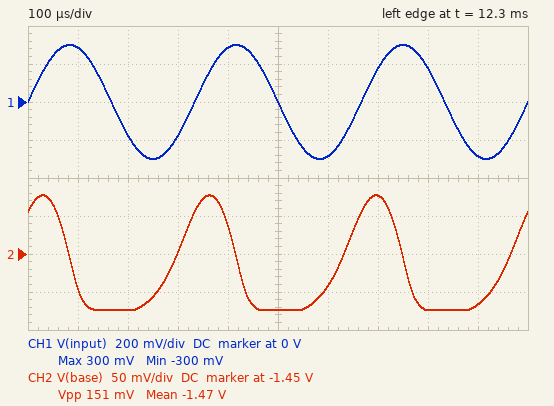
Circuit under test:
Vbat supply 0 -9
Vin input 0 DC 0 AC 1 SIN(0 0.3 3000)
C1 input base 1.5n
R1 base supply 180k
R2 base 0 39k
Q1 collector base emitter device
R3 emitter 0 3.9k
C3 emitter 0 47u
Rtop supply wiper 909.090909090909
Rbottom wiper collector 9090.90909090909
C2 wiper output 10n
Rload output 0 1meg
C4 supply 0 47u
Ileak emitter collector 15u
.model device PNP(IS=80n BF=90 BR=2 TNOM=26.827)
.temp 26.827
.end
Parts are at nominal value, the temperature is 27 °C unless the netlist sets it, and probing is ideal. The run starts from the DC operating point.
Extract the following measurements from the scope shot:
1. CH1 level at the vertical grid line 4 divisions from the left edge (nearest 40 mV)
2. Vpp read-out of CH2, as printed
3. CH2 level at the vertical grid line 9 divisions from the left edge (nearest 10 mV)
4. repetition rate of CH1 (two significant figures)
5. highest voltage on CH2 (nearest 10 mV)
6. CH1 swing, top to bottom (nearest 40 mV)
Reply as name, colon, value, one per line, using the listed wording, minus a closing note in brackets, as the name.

CH1 level at the vertical grid line 4 divisions from the left edge: 280 mV
Vpp read-out of CH2, as printed: 151 mV
CH2 level at the vertical grid line 9 divisions from the left edge: -1.52 V
repetition rate of CH1: 3.0 kHz
highest voltage on CH2: -1.37 V
CH1 swing, top to bottom: 600 mV
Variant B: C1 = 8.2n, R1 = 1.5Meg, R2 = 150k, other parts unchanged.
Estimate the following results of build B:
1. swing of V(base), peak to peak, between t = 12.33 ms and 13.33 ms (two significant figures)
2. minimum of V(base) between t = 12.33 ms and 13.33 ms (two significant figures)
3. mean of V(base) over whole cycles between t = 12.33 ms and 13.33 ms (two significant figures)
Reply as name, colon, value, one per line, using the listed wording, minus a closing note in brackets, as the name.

swing of V(base), peak to peak, between t = 12.33 ms and 13.33 ms: 560 mV
minimum of V(base) between t = 12.33 ms and 13.33 ms: -730 mV
mean of V(base) over whole cycles between t = 12.33 ms and 13.33 ms: -460 mV
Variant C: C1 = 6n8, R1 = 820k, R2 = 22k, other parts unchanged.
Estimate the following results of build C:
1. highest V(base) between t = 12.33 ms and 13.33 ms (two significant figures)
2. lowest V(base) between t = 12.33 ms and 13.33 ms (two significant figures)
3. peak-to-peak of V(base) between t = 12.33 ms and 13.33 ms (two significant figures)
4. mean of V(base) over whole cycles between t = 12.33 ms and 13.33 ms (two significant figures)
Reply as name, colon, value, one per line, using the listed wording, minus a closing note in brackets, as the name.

highest V(base) between t = 12.33 ms and 13.33 ms: 96 mV
lowest V(base) between t = 12.33 ms and 13.33 ms: -400 mV
peak-to-peak of V(base) between t = 12.33 ms and 13.33 ms: 490 mV
mean of V(base) over whole cycles between t = 12.33 ms and 13.33 ms: -170 mV
